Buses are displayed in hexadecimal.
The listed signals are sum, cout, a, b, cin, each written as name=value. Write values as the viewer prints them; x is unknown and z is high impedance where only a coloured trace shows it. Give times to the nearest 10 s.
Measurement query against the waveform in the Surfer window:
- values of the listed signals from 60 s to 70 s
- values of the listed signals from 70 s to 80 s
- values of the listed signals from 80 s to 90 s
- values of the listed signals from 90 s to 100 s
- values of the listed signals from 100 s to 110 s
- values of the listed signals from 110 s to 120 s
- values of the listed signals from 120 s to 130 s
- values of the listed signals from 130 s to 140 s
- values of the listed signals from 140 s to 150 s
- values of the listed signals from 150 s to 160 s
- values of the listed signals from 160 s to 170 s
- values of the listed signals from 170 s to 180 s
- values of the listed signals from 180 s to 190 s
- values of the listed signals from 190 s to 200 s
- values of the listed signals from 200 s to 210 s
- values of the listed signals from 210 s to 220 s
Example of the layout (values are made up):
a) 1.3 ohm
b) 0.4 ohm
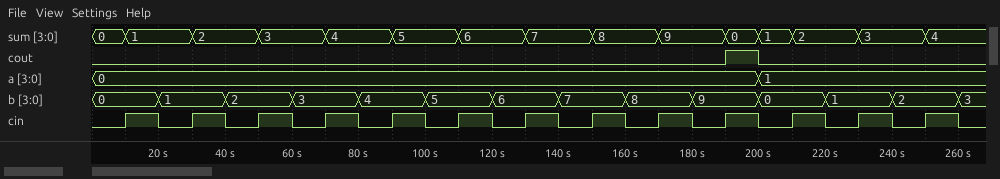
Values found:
a) sum=3, cout=0, a=0, b=3, cin=0
b) sum=4, cout=0, a=0, b=3, cin=1
c) sum=4, cout=0, a=0, b=4, cin=0
d) sum=5, cout=0, a=0, b=4, cin=1
e) sum=5, cout=0, a=0, b=5, cin=0
f) sum=6, cout=0, a=0, b=5, cin=1
g) sum=6, cout=0, a=0, b=6, cin=0
h) sum=7, cout=0, a=0, b=6, cin=1
i) sum=7, cout=0, a=0, b=7, cin=0
j) sum=8, cout=0, a=0, b=7, cin=1
k) sum=8, cout=0, a=0, b=8, cin=0
l) sum=9, cout=0, a=0, b=8, cin=1
m) sum=9, cout=0, a=0, b=9, cin=0
n) sum=0, cout=1, a=0, b=9, cin=1
o) sum=1, cout=0, a=1, b=0, cin=0
p) sum=2, cout=0, a=1, b=0, cin=1
